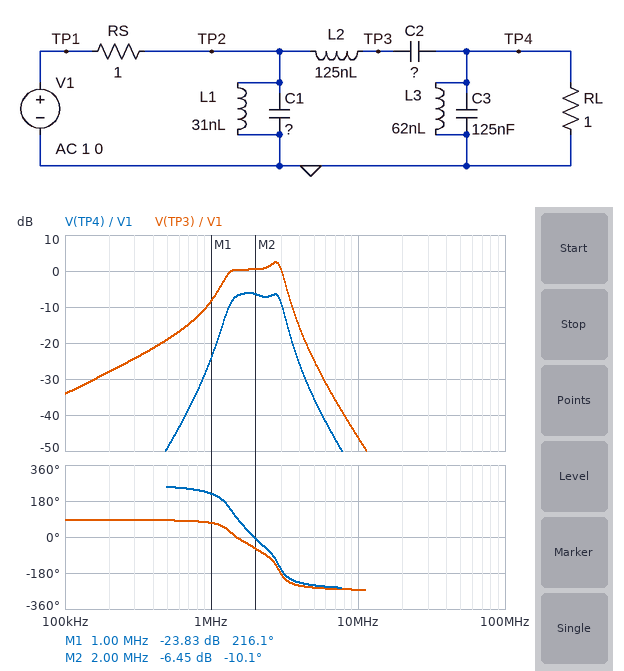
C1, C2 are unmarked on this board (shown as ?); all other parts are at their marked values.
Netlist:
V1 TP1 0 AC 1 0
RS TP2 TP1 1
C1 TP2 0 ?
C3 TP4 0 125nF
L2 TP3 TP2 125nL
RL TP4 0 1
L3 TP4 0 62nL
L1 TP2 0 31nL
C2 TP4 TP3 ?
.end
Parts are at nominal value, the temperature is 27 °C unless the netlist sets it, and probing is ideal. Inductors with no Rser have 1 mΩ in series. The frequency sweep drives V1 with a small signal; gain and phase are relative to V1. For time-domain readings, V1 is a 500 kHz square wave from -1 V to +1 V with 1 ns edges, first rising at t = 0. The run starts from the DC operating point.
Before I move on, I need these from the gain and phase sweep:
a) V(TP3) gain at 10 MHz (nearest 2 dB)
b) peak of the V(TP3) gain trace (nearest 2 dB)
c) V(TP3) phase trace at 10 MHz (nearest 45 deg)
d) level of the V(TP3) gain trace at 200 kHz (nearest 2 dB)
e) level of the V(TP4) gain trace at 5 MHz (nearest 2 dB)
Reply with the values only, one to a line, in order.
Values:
-46 dB
2 dB
-270 deg
-28 dB
-36 dB
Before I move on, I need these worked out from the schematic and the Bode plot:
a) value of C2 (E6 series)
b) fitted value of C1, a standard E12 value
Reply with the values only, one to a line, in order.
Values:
47 nF
220 nF
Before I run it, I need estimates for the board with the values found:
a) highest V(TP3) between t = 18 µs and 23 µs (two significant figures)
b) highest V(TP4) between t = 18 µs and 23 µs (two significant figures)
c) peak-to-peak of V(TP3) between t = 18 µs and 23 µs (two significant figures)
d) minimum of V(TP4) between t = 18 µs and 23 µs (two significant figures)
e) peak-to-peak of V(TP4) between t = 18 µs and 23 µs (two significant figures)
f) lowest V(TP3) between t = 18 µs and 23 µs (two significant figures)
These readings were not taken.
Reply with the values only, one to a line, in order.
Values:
880 mV
310 mV
1.8 V
-310 mV
630 mV
-880 mV
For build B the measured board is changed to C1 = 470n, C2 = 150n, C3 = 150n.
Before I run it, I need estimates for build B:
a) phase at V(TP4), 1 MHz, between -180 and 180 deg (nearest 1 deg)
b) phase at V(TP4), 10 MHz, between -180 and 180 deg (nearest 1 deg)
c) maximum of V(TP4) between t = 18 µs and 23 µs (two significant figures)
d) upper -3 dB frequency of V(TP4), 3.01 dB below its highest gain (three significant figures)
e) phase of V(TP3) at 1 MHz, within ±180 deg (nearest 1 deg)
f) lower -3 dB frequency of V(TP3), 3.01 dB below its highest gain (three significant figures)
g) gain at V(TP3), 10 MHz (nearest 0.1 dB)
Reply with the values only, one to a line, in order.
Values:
73 deg
98 deg
220 mV
1.76 MHz
-51 deg
761 kHz
-60.3 dB
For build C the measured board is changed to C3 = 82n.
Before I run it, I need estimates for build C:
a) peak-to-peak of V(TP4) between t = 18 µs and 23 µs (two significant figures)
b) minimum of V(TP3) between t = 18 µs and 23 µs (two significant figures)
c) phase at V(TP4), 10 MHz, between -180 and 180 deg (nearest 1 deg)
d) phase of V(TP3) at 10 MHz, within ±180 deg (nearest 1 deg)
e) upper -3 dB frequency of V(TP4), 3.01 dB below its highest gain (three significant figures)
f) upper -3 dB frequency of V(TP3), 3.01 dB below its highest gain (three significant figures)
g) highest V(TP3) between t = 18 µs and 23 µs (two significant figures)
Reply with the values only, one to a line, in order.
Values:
660 mV
-910 mV
106 deg
99 deg
2.96 MHz
2.07 MHz
910 mV
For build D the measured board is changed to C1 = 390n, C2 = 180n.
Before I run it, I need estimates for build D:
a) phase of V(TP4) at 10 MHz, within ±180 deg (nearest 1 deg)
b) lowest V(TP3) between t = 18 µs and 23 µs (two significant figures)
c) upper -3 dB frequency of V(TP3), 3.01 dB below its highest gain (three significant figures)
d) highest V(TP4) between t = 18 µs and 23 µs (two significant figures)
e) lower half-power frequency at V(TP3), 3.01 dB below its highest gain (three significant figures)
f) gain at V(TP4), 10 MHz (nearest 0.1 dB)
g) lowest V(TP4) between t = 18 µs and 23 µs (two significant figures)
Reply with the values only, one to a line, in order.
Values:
100 deg
-380 mV
819 kHz
240 mV
718 kHz
-62.9 dB
-240 mV
